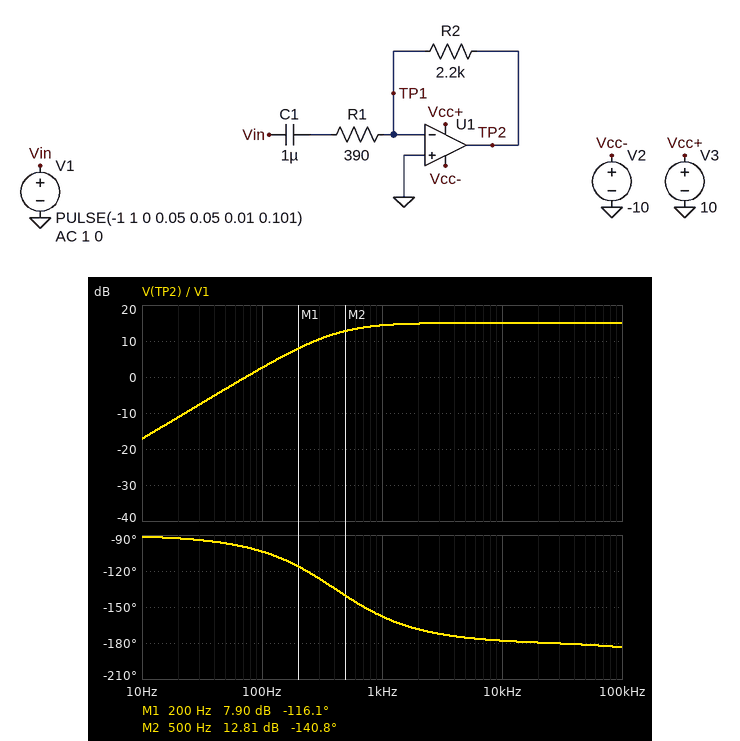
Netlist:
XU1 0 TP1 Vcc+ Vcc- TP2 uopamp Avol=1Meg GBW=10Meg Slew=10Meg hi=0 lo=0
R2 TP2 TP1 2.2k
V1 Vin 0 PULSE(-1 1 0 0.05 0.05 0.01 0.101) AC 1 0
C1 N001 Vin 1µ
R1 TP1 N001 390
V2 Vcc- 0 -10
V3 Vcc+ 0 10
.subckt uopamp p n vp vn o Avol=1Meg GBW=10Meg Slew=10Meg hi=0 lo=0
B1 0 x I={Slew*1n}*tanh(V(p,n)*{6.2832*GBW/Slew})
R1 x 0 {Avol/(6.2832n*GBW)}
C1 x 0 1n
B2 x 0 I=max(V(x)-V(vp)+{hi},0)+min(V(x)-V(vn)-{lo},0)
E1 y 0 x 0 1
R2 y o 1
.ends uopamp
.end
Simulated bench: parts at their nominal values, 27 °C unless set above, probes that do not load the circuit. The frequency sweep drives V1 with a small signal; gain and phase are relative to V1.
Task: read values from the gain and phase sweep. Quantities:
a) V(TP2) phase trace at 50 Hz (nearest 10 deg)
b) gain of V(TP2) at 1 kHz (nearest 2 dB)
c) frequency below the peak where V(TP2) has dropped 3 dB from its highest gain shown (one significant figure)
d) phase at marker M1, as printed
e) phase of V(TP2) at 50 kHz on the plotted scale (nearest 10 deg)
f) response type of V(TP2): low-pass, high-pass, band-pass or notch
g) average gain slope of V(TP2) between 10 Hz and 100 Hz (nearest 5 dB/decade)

-100 deg
14 dB
400 Hz
-116.1 deg
-180 deg
high-pass
20 dB/decade
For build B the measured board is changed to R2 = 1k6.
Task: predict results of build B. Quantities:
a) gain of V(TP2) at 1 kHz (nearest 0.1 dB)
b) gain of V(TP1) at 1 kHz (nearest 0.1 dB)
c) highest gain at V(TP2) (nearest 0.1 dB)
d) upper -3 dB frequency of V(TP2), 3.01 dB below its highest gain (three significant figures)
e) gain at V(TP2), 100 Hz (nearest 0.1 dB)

11.6 dB
-68.4 dB
12.3 dB
1.96 MHz
-0.2 dB
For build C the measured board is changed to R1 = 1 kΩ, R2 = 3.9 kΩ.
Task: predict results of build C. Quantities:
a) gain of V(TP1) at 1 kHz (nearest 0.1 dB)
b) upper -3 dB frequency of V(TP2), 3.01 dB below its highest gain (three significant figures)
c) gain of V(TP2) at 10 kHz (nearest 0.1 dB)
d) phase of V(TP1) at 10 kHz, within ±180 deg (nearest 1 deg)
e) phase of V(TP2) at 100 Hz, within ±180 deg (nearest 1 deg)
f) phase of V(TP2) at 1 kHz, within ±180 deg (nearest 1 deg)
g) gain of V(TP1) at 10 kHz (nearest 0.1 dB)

-68.3 dB
2.04 MHz
11.8 dB
91 deg
-122 deg
-171 deg
-48.2 dB
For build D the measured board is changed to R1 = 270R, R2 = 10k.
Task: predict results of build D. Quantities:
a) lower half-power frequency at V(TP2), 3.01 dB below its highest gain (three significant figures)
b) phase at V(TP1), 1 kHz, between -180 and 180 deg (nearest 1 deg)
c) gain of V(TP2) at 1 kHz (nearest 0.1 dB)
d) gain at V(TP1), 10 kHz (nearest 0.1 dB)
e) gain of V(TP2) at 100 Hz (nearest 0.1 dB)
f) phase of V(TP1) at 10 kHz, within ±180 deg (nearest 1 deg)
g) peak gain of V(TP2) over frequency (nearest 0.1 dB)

588 Hz
120 deg
30.1 dB
-28.6 dB
15.8 dB
91 deg
31.4 dB
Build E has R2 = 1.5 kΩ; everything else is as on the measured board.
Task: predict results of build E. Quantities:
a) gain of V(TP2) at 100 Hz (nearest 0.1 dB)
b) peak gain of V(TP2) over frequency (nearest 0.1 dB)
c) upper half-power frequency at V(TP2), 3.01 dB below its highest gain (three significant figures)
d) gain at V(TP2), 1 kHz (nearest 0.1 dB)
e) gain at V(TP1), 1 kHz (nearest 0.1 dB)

-0.8 dB
11.7 dB
2.06 MHz
11.0 dB
-69.0 dB
